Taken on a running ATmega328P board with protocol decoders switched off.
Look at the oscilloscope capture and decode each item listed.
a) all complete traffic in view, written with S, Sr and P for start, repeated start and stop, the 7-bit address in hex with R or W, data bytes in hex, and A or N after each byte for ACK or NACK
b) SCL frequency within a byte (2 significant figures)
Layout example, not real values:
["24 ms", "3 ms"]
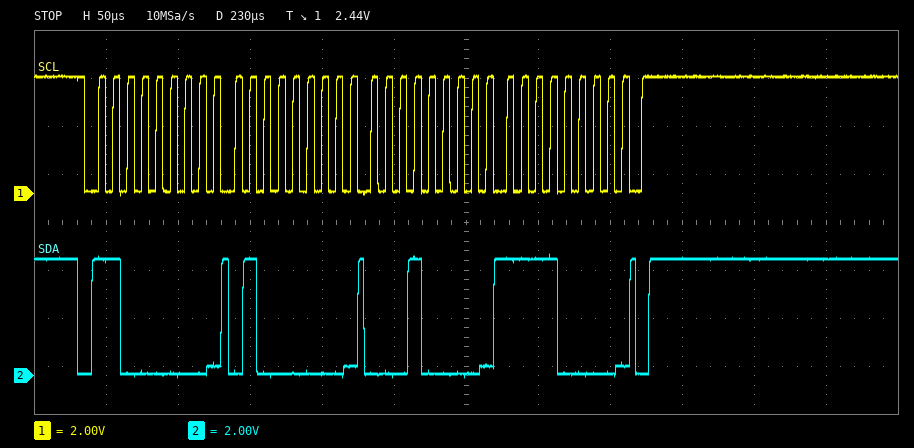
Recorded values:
["S 60W A 40 A 10 A F0 A P", "100 kHz"]
